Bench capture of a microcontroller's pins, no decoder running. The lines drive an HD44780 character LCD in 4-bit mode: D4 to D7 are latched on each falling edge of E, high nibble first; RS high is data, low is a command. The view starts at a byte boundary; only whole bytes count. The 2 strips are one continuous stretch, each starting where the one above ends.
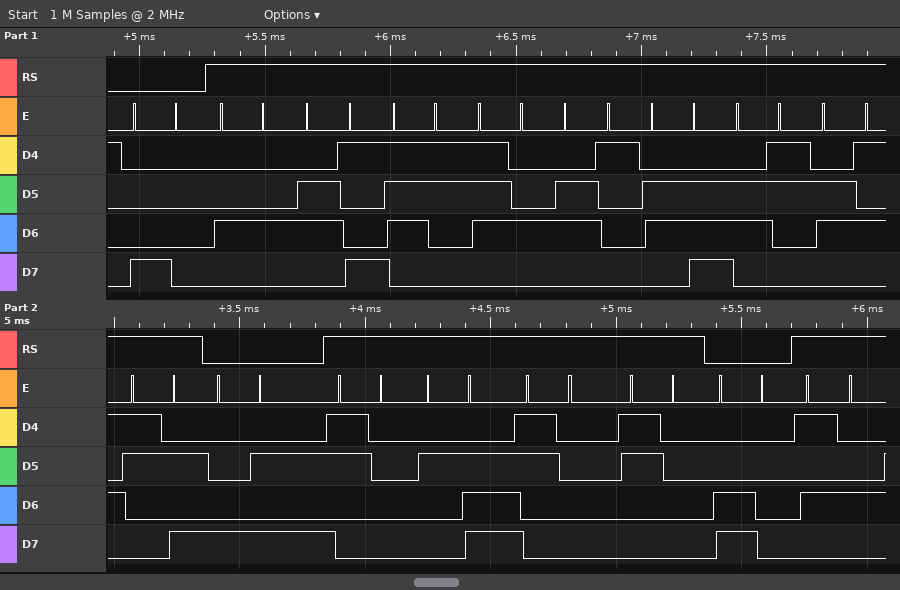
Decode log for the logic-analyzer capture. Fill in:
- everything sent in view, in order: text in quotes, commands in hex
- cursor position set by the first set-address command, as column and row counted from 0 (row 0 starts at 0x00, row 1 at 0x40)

0x80 "Distance:" 0x8A "0.00" 0xC0 "T"
column 0, row 0
